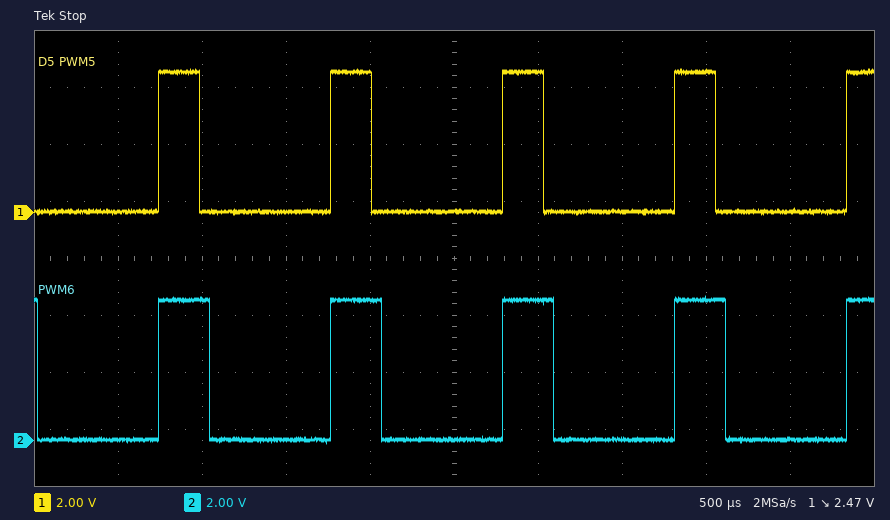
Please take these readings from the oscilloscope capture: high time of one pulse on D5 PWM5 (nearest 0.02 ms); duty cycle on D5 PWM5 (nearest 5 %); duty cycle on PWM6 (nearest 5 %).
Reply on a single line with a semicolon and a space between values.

0.24 ms; 25 %; 30 %
